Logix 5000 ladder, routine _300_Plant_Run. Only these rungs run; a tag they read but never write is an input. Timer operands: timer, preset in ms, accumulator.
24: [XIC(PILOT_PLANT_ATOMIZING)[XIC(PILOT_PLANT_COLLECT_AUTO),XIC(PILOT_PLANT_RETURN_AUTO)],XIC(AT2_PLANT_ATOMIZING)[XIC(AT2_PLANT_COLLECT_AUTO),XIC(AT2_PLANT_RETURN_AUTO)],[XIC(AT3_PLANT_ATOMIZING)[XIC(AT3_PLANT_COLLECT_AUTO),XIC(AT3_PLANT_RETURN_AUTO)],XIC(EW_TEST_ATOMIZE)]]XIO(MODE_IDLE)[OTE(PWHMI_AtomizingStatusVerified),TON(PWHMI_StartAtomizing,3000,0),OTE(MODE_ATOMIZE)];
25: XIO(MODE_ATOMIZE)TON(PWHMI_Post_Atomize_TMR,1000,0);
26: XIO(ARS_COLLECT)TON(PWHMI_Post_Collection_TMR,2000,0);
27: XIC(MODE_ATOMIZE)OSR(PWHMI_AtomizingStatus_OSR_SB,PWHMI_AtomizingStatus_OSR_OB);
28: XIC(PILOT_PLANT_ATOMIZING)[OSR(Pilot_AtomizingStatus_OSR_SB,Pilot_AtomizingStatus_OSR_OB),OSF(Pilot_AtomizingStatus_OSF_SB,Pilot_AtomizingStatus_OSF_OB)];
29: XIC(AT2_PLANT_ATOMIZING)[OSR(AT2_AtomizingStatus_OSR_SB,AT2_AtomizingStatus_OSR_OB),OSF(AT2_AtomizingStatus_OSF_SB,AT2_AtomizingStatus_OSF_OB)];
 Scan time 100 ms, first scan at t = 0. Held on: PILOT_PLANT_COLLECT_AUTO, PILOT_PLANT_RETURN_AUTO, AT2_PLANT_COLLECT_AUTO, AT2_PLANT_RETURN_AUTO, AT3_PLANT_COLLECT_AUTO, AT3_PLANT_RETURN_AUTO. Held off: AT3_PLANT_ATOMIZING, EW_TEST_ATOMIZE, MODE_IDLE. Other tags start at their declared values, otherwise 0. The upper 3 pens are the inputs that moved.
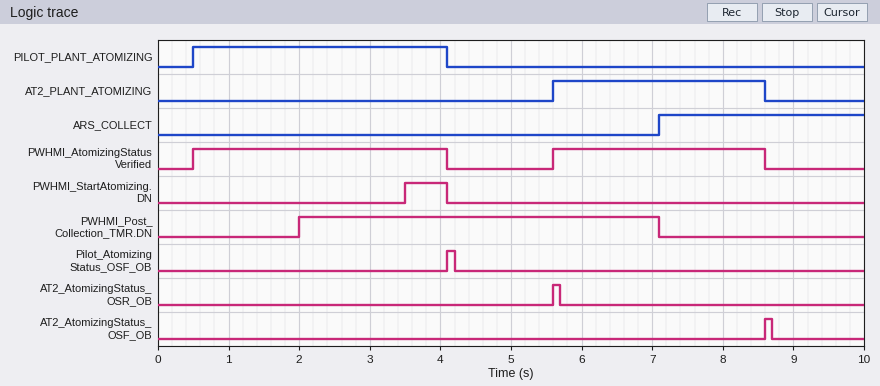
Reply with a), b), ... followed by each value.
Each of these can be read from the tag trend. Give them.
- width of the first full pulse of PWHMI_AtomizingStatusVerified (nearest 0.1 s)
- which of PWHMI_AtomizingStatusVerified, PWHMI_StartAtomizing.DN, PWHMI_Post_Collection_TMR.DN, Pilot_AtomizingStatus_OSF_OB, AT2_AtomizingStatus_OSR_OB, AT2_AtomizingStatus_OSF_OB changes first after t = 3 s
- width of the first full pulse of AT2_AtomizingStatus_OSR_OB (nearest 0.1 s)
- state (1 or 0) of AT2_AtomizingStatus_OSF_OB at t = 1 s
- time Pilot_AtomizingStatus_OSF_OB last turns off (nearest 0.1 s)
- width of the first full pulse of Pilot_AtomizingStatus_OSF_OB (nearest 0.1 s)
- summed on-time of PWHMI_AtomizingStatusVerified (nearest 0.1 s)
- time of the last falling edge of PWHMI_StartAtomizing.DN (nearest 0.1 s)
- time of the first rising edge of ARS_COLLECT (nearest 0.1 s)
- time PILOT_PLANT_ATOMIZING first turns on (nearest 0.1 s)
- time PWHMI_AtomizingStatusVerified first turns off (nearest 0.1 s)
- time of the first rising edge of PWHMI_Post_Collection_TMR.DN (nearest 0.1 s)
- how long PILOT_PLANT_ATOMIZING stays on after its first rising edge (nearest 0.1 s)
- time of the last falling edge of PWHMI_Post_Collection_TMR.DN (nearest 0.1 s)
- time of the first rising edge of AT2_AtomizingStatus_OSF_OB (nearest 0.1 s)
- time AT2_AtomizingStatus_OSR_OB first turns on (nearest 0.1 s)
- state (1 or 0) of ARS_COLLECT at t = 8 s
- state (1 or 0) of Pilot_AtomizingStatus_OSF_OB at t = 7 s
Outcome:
a) 3.6 s
b) PWHMI_StartAtomizing.DN
c) 0.1 s
d) 0
e) 4.2 s
f) 0.1 s
g) 6.6 s
h) 4.1 s
i) 7.1 s
j) 0.5 s
k) 4.1 s
l) 2.0 s
m) 3.6 s
n) 7.1 s
o) 8.6 s
p) 5.6 s
q) 1
r) 0
